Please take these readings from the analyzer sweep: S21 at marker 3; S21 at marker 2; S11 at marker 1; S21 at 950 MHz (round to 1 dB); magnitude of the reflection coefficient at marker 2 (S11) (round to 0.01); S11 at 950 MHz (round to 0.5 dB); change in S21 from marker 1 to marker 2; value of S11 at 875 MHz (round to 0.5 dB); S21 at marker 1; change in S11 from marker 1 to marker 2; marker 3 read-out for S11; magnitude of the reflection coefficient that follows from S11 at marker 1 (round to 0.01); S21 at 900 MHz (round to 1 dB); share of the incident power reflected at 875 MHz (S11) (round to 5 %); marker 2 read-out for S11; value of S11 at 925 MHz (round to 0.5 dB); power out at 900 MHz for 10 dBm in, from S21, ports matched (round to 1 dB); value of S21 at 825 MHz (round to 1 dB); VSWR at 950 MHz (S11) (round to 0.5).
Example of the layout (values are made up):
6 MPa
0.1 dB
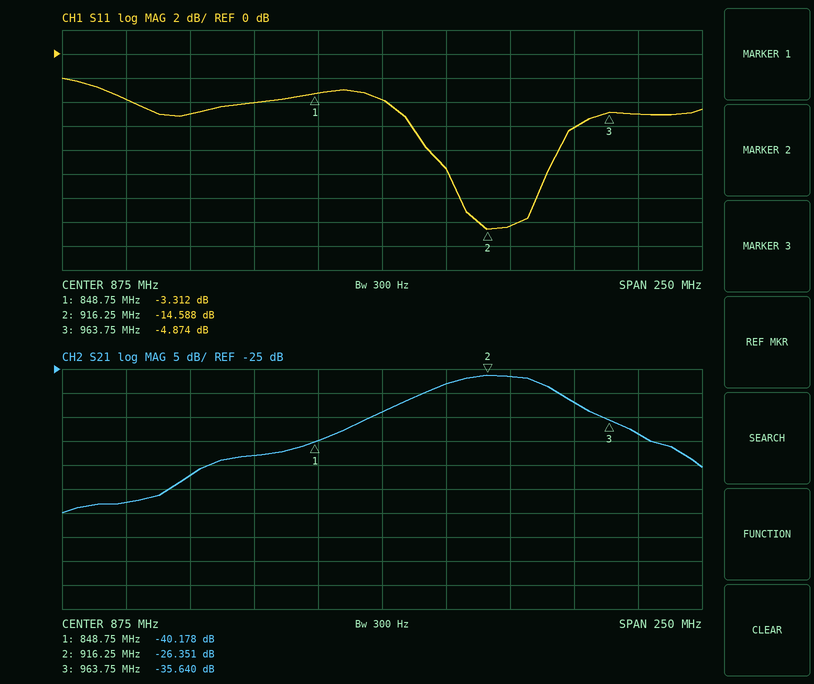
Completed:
-35.640 dB
-26.351 dB
-3.312 dB
-32 dB
0.19
-6.0 dB
13.827 dB
-4.0 dB
-40.178 dB
-11.276 dB
-4.874 dB
0.68
-28 dB
40 %
-14.588 dB
-14.5 dB
-18 dBm
-43 dB
3.0
